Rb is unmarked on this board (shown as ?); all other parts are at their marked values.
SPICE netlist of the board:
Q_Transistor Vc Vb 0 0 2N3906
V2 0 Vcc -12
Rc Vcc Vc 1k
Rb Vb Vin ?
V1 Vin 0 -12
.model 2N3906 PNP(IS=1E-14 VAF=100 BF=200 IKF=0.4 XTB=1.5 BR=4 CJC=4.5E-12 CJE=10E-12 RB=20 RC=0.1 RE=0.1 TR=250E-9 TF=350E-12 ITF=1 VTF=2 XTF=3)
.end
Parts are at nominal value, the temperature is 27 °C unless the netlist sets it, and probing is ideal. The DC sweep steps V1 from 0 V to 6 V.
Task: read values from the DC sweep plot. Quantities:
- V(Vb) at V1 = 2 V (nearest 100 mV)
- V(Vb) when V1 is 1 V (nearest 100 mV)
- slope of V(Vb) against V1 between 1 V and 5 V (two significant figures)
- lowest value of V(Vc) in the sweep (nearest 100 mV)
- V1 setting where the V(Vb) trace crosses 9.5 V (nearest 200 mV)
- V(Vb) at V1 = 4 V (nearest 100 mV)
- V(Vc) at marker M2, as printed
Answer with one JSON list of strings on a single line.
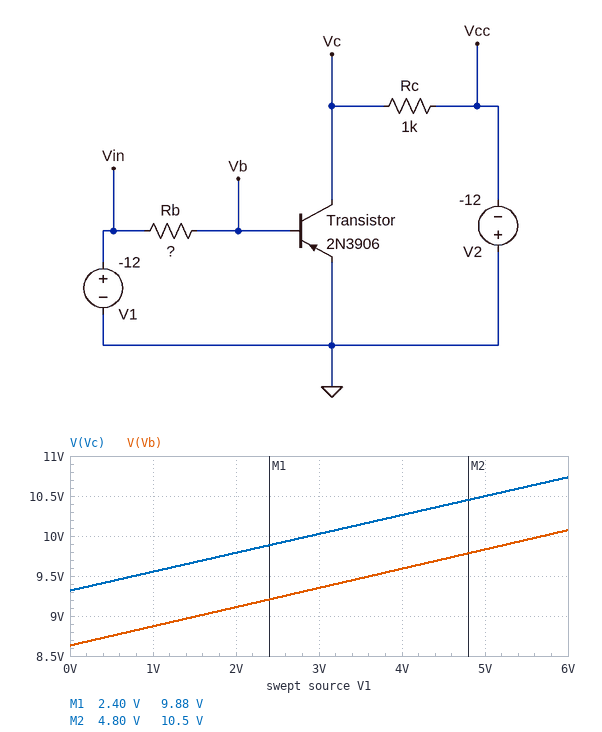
["9.1 V", "8.9 V", "0.24 V/V", "9.3 V", "3.6 V", "9.6 V", "10.5 V"]
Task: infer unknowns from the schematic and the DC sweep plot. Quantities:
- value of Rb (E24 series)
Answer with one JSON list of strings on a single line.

["16 kΩ"]
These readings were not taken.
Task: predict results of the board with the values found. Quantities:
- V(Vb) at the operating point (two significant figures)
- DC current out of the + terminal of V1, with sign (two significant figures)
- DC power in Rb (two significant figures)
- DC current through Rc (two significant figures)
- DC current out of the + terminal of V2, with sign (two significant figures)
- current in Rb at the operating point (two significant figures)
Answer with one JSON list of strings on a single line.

["5.8 V", "-1.1 mA", "20 mW", "5.5 mA", "-5.5 mA", "1.1 mA"]
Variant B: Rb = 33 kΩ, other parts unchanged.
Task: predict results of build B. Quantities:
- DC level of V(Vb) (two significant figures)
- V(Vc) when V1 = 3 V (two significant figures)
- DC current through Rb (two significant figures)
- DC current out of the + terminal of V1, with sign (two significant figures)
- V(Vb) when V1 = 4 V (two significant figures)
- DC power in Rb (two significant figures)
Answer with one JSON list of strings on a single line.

["8.3 V", "11 V", "610 µA", "-610 µA", "10 V", "12 mW"]
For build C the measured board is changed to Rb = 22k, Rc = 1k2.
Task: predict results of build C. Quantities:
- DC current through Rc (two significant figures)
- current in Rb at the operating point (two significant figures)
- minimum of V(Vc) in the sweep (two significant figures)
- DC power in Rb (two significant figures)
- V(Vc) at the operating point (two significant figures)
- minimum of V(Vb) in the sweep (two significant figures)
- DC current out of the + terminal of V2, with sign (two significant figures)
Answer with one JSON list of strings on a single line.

["4.1 mA", "830 µA", "9.6 V", "15 mW", "7.0 V", "8.9 V", "-4.1 mA"]
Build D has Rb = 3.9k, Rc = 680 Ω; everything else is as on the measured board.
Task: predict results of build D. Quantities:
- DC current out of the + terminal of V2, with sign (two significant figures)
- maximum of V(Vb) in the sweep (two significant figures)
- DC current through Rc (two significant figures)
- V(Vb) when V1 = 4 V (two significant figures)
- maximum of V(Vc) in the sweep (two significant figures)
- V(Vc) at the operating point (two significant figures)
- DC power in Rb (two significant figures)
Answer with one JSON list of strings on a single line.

["-16 mA", "8.8 V", "16 mA", "7.9 V", "9.5 V", "1.2 V", "40 mW"]
